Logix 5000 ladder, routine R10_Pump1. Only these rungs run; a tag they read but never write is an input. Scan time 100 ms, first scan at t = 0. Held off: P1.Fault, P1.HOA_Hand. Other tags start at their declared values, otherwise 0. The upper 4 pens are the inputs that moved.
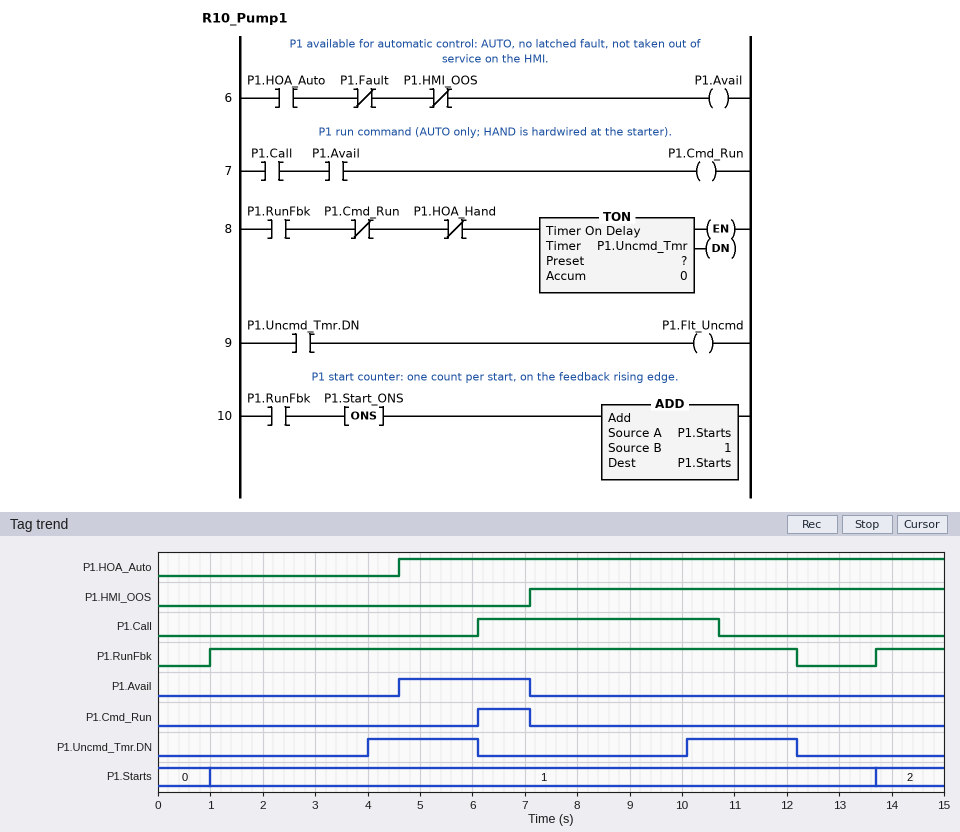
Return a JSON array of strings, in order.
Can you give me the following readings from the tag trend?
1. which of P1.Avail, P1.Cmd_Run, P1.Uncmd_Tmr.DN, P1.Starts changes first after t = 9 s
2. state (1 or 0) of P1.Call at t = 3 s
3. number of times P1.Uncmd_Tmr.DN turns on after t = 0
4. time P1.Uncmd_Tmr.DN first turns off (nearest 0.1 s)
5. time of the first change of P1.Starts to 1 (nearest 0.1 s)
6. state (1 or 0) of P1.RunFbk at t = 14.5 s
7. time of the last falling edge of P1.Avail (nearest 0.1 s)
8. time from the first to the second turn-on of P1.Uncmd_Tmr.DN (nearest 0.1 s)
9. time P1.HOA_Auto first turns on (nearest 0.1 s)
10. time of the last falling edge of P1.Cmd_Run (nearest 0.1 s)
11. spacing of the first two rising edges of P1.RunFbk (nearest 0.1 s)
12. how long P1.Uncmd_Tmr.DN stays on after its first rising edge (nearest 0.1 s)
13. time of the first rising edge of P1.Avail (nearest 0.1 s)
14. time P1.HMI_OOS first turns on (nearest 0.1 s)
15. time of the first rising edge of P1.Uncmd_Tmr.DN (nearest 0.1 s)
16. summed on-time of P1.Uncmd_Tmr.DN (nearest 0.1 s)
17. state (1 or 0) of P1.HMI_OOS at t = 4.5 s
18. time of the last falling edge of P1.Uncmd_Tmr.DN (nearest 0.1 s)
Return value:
["P1.Uncmd_Tmr.DN", "0", "2", "6.1 s", "1.0 s", "1", "7.1 s", "6.1 s", "4.6 s", "7.1 s", "12.7 s", "2.1 s", "4.6 s", "7.1 s", "4.0 s", "4.2 s", "0", "12.2 s"]
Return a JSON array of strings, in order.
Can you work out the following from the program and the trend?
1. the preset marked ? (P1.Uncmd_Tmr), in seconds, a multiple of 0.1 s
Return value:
["3.0 s"]
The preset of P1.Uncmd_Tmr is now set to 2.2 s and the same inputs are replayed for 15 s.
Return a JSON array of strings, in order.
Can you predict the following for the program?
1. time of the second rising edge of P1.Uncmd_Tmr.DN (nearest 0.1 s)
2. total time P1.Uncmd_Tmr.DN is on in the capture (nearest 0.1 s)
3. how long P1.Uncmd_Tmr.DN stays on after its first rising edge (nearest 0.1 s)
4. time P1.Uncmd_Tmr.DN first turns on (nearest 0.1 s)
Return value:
["9.3 s", "5.8 s", "2.9 s", "3.2 s"]
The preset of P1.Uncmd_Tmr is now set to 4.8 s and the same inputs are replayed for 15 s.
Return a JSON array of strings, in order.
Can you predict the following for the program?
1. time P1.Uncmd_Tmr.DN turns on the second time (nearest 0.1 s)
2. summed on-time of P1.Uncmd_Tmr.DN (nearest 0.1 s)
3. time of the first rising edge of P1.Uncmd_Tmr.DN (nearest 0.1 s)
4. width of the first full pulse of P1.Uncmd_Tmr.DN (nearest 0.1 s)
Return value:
["11.9 s", "0.6 s", "5.8 s", "0.3 s"]
